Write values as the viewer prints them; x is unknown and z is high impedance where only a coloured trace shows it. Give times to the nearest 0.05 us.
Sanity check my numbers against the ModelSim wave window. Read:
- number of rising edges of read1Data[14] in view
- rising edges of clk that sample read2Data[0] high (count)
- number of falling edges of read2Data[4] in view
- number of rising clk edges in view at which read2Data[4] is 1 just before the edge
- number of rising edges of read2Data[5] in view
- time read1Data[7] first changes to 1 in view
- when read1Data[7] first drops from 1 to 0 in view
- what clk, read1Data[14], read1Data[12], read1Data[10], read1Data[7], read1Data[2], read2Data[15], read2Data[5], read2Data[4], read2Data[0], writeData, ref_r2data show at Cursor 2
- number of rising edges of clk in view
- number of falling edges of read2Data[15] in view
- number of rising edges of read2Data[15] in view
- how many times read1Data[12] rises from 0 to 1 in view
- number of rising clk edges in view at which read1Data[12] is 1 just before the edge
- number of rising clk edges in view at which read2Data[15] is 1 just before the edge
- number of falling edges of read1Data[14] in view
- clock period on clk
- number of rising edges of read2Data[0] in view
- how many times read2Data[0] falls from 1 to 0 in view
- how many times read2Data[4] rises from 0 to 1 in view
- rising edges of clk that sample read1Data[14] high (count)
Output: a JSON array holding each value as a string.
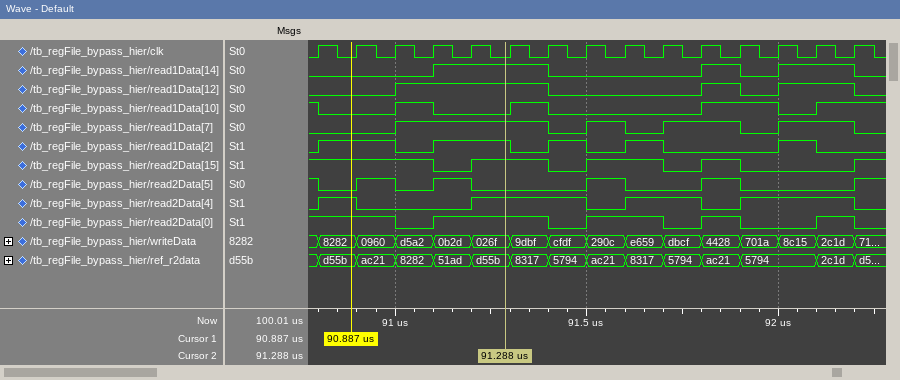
["3", "10", "4", "9", "5", "91 us", "91.4 us", "clk=0, read1Data[14]=1, read1Data[12]=1, read1Data[10]=0, read1Data[7]=1, read1Data[2]=1, read2Data[15]=1, read2Data[5]=0, read2Data[4]=1, read2Data[0]=1, writeData=026f, ref_r2data=d55b", "15", "4", "4", "3", "7", "9", "3", "0.1 us", "4", "5", "4", "6"]
